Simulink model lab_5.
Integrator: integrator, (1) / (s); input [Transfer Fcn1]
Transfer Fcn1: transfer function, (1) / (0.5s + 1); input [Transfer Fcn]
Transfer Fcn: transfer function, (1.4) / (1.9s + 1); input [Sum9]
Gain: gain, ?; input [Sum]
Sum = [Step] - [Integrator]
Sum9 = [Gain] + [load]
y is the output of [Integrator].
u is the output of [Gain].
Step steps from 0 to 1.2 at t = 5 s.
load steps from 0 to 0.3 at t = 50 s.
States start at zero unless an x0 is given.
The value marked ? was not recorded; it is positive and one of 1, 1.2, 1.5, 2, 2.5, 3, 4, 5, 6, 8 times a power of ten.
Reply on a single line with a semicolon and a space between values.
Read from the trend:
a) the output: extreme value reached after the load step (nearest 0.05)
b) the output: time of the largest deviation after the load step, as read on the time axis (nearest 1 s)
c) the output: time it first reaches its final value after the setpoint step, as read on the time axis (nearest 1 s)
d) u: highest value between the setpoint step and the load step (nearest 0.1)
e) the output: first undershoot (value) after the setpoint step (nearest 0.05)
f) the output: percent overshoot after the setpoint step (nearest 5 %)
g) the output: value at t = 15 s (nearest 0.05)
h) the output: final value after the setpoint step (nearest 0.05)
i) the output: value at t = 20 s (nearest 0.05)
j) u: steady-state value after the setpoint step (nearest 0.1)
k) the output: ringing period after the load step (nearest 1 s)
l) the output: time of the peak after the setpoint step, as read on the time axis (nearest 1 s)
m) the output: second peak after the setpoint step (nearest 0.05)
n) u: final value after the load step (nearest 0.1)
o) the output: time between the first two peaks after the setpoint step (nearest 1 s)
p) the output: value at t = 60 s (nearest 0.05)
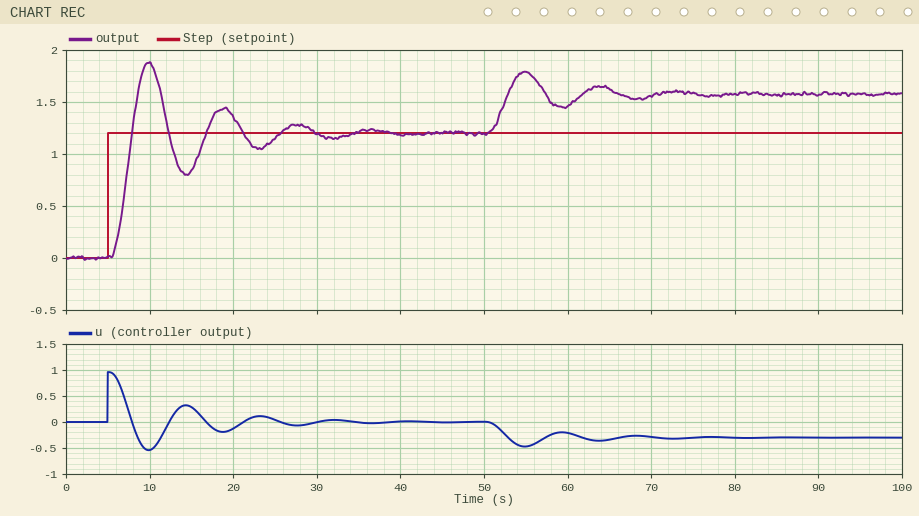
1.80; 55 s; 8 s; 1.0; 0.80; 55 %; 0.85; 1.20; 1.35; 0.0; 9 s; 10 s; 1.45; -0.3; 9 s; 1.45
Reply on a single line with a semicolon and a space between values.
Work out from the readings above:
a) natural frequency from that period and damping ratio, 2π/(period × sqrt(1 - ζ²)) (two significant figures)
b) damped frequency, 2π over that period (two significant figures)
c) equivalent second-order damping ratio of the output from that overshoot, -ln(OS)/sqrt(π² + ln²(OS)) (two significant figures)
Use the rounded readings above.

0.71 rad/s; 0.70 rad/s; 0.19
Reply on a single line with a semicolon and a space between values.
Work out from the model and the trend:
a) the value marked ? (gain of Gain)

0.8
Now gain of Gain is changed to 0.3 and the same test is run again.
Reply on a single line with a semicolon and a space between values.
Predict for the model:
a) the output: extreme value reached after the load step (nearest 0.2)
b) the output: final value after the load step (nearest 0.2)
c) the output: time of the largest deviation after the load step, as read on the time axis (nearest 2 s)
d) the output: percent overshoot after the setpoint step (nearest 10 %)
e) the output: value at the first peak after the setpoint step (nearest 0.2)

2.4; 2.2; 58 s; 20 %; 1.4
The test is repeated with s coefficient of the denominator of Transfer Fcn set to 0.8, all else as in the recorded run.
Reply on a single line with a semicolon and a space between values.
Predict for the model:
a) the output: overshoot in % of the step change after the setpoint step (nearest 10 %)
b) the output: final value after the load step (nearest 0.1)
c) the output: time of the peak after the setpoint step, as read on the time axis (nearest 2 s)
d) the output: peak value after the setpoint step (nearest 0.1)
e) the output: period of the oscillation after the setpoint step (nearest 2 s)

40 %; 1.6; 8 s; 1.7; 6 s
